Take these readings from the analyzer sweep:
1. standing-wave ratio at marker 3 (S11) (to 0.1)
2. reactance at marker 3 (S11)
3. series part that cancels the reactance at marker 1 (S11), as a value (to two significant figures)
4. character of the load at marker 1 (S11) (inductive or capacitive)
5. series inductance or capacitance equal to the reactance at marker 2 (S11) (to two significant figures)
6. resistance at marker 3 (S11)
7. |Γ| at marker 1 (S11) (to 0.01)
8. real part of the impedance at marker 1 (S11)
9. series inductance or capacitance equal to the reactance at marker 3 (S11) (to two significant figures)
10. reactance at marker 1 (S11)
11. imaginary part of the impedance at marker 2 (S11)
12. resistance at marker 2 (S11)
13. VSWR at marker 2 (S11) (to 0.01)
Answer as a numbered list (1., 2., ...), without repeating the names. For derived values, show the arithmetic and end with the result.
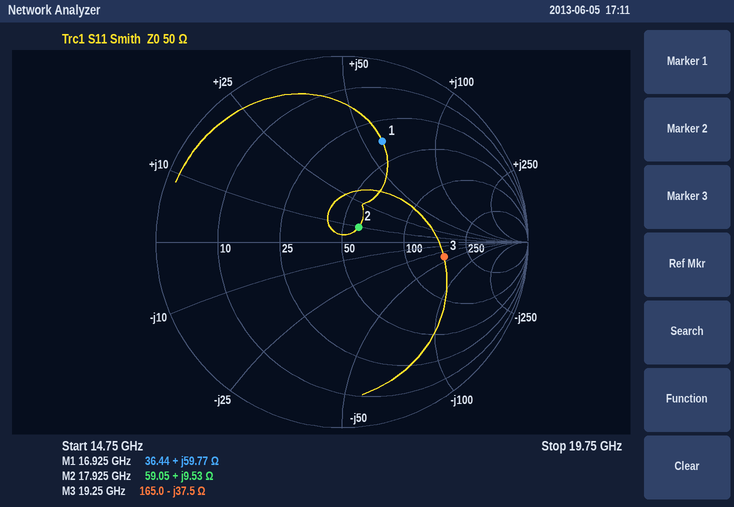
1. 3.5
2. -37.5 Ω
3. C = 1/(2π × 16.925 GHz × 59.77 Ω) ≈ 157 fF, so 160 fF to two significant figures
4. inductive
5. L = 9.53 Ω/(2π × 17.925 GHz) ≈ 85 pH
6. 165.0 Ω
7. 0.58
8. 36.44 Ω
9. C = 1/(2π × 19.25 GHz × 37.5 Ω) ≈ 220 fF
10. +59.77 Ω
11. +9.53 Ω
12. 59.05 Ω
13. 1.27
